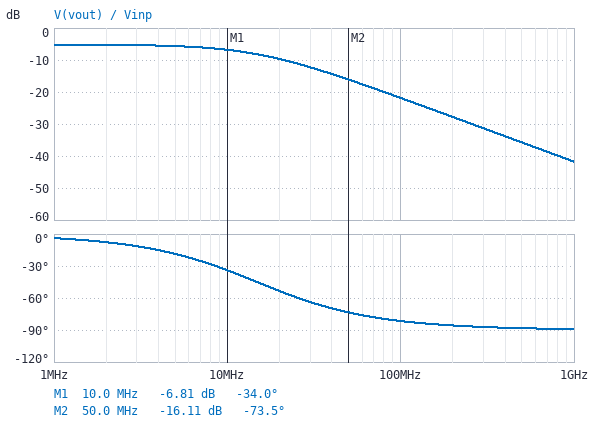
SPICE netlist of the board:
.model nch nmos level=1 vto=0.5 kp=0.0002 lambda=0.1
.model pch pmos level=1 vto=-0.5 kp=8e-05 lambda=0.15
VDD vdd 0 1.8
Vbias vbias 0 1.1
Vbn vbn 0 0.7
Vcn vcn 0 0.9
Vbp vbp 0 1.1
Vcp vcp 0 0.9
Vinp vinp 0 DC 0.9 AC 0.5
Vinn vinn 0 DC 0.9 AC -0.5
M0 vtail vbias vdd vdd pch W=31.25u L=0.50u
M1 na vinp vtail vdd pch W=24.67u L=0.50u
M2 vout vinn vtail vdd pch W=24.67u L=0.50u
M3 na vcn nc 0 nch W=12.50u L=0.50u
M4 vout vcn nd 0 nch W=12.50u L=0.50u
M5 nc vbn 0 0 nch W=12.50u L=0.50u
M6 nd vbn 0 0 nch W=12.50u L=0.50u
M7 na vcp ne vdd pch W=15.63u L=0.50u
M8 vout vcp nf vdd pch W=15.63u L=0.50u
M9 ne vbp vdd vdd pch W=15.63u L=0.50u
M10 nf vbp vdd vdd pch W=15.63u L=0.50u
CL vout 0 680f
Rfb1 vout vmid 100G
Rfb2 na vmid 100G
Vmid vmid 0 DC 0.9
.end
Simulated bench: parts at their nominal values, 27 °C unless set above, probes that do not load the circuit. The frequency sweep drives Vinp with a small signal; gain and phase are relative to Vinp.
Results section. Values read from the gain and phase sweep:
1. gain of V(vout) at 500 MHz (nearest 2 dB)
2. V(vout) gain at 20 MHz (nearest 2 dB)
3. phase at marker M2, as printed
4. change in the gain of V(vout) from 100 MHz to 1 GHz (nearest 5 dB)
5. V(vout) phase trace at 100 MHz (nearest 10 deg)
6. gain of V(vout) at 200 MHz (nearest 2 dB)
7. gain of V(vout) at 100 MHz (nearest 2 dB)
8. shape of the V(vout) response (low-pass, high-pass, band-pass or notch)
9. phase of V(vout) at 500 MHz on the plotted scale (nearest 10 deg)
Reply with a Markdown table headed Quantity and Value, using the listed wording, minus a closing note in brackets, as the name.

| Quantity | Value |
|---|---|
| gain of V(vout) at 500 MHz | -36 dB |
| V(vout) gain at 20 MHz | -10 dB |
| phase at marker M2, as printed | -73.5 deg |
| change in the gain of V(vout) from 100 MHz to 1 GHz | -20 dB |
| V(vout) phase trace at 100 MHz | -80 deg |
| gain of V(vout) at 200 MHz | -28 dB |
| gain of V(vout) at 100 MHz | -22 dB |
| shape of the V(vout) response | low-pass |
| phase of V(vout) at 500 MHz on the plotted scale | -90 deg |
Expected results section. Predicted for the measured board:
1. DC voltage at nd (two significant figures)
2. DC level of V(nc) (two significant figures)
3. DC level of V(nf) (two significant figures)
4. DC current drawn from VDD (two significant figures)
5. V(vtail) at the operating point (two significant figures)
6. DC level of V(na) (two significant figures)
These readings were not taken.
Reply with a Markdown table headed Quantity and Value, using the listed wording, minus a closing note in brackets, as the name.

| Quantity | Value |
|---|---|
| DC voltage at nd | 210 mV |
| DC level of V(nc) | 210 mV |
| DC level of V(nf) | 1.6 V |
| DC current drawn from VDD | 200 µA |
| V(vtail) at the operating point | 1.6 V |
| DC level of V(na) | 1.5 V |
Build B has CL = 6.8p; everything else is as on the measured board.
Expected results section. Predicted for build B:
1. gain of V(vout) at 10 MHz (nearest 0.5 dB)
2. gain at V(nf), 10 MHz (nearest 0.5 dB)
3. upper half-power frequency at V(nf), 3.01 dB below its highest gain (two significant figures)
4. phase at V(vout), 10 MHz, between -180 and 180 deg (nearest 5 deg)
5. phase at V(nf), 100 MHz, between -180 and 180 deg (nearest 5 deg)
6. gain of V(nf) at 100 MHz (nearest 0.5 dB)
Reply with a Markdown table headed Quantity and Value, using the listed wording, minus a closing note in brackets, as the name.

| Quantity | Value |
|---|---|
| gain of V(vout) at 10 MHz | -22.0 dB |
| gain at V(nf), 10 MHz | -29.5 dB |
| upper half-power frequency at V(nf), 3.01 dB below its highest gain | 1.5 MHz |
| phase at V(vout), 10 MHz, between -180 and 180 deg | -80 deg |
| phase at V(nf), 100 MHz, between -180 and 180 deg | -90 deg |
| gain of V(nf) at 100 MHz | -49.5 dB |
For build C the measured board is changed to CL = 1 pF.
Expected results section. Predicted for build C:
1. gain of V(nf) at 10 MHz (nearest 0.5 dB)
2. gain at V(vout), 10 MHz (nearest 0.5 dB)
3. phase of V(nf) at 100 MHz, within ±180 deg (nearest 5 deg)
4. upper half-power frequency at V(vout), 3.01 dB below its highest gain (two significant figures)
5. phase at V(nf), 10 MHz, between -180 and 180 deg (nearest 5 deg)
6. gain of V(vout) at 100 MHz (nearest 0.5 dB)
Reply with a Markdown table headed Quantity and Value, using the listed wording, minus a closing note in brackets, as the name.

| Quantity | Value |
|---|---|
| gain of V(nf) at 10 MHz | -15.5 dB |
| gain at V(vout), 10 MHz | -8.0 dB |
| phase of V(nf) at 100 MHz, within ±180 deg | -85 deg |
| upper half-power frequency at V(vout), 3.01 dB below its highest gain | 10 MHz |
| phase at V(nf), 10 MHz, between -180 and 180 deg | -45 deg |
| gain of V(vout) at 100 MHz | -25.0 dB |
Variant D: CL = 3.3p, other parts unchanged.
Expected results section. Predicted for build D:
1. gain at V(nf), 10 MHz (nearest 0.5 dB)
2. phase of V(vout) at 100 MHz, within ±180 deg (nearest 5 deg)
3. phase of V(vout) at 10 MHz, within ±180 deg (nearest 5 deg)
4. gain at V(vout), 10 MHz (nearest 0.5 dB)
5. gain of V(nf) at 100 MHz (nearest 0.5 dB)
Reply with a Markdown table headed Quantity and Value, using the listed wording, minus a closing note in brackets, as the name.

| Quantity | Value |
|---|---|
| gain at V(nf), 10 MHz | -23.5 dB |
| phase of V(vout) at 100 MHz, within ±180 deg | -90 deg |
| phase of V(vout) at 10 MHz, within ±180 deg | -75 deg |
| gain at V(vout), 10 MHz | -16.0 dB |
| gain of V(nf) at 100 MHz | -43.0 dB |
